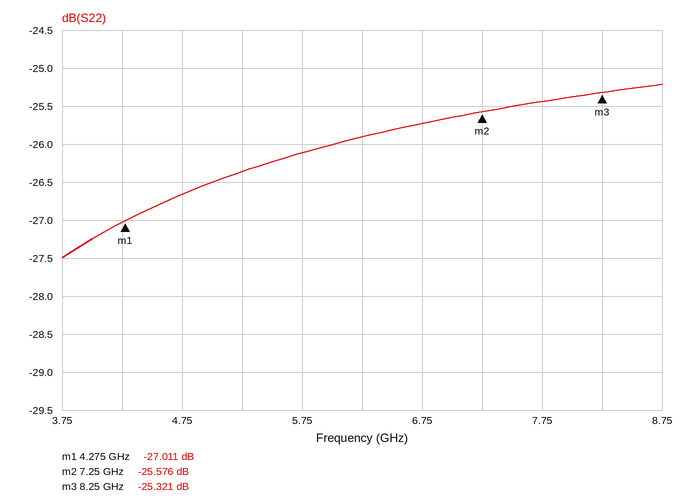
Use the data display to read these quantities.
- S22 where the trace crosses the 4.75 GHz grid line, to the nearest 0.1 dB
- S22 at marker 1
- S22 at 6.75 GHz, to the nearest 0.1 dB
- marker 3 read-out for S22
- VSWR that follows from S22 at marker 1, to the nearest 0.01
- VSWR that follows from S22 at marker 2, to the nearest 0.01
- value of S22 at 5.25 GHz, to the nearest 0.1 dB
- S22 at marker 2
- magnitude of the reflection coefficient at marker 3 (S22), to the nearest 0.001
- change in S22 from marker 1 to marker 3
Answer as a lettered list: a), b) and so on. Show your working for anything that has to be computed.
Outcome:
a) -26.7 dB
b) -27.011 dB
c) -25.7 dB
d) -25.321 dB
e) (1 + 0.0446)/(1 − 0.0446) ≈ 1.09
f) (1 + 0.0526)/(1 − 0.0526) ≈ 1.11
g) -26.4 dB
h) -25.576 dB
i) 10^(-25.321/20) ≈ 0.054
j) -25.321 − (-27.011) = 1.690 dB
